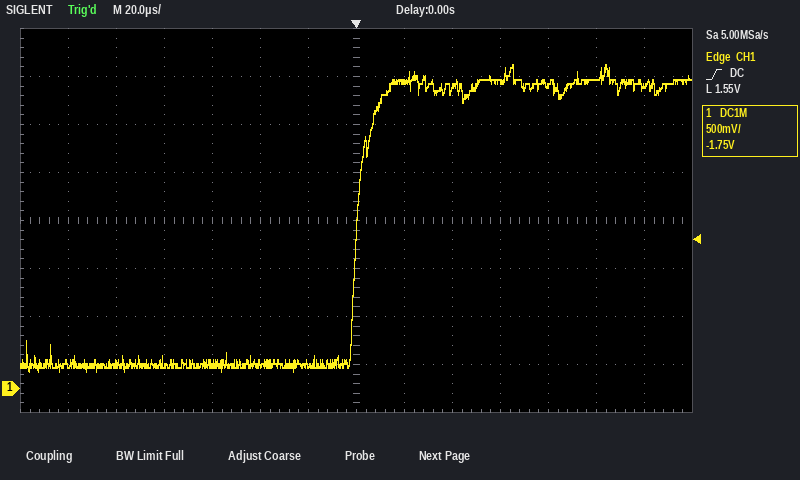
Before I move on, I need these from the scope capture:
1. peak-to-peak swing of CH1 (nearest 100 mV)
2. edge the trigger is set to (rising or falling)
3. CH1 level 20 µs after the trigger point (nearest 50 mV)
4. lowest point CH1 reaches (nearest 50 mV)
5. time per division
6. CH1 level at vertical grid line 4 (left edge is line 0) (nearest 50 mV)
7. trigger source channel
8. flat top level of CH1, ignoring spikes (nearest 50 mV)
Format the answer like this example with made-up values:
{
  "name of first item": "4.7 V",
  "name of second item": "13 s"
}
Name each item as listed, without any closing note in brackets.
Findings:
{
  "peak-to-peak swing of CH1": "3.20 V",
  "edge the trigger is set to": "rising",
  "CH1 level 20 µs after the trigger point": "3.20 V",
  "lowest point CH1 reaches": "200 mV",
  "time per division": "20 µs",
  "CH1 level at vertical grid line 4 (left edge is line 0)": "250 mV",
  "trigger source channel": "CH1",
  "flat top level of CH1, ignoring spikes": "3.20 V"
}
